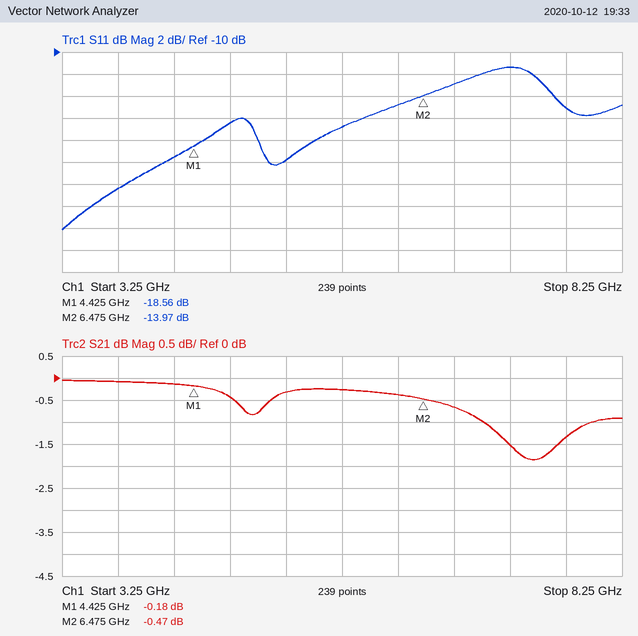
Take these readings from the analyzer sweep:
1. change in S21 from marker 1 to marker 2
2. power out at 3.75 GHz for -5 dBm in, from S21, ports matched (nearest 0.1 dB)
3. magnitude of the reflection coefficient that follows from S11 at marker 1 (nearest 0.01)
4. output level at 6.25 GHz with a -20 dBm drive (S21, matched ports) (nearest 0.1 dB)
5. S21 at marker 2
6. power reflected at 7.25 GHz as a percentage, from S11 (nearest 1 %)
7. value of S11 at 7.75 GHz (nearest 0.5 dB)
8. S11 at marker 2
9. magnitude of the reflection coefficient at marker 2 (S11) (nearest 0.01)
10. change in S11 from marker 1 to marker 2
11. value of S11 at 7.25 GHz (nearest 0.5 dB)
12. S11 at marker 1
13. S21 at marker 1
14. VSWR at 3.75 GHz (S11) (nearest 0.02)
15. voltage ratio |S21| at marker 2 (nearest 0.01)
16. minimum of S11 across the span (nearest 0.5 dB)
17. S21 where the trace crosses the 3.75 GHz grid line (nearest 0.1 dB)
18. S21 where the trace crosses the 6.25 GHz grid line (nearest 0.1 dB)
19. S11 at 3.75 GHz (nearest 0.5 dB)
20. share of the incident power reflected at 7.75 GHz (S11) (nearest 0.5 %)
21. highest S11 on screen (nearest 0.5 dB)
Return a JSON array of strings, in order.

["-0.29 dB", "-5.1 dBm", "0.12", "-20.4 dBm", "-0.47 dB", "7 %", "-15.0 dB", "-13.97 dB", "0.20", "4.59 dB", "-11.5 dB", "-18.56 dB", "-0.18 dB", "1.16", "0.95", "-26.0 dB", "-0.1 dB", "-0.4 dB", "-22.5 dB", "3.0 %", "-11.5 dB"]
